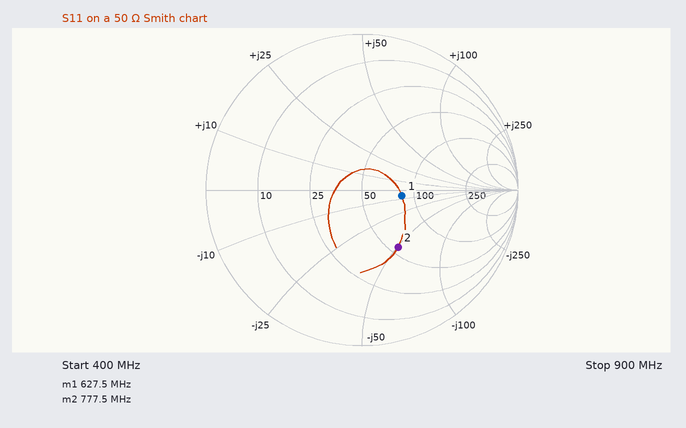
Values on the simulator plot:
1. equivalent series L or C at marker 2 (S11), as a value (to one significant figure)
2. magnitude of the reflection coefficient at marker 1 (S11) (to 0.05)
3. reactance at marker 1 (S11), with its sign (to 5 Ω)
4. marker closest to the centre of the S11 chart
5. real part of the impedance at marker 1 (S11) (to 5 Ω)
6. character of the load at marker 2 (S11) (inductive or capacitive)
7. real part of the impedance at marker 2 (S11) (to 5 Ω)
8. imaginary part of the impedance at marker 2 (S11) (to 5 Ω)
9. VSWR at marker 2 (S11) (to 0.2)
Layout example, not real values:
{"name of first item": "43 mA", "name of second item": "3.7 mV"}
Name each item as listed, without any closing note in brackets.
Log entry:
{"equivalent series L or C at marker 2 (S11), as a value": "4 pF", "magnitude of the reflection coefficient at marker 1 (S11)": "0.25", "reactance at marker 1 (S11), with its sign": "-5 Ω", "marker closest to the centre of the S11 chart": "marker 1", "real part of the impedance at marker 1 (S11)": "85 Ω", "character of the load at marker 2 (S11)": "capacitive", "real part of the impedance at marker 2 (S11)": "55 Ω", "imaginary part of the impedance at marker 2 (S11)": "-50 Ω", "VSWR at marker 2 (S11)": "2.6"}
